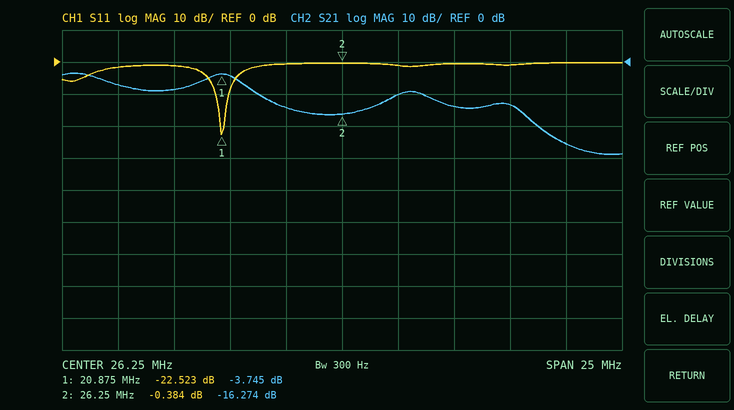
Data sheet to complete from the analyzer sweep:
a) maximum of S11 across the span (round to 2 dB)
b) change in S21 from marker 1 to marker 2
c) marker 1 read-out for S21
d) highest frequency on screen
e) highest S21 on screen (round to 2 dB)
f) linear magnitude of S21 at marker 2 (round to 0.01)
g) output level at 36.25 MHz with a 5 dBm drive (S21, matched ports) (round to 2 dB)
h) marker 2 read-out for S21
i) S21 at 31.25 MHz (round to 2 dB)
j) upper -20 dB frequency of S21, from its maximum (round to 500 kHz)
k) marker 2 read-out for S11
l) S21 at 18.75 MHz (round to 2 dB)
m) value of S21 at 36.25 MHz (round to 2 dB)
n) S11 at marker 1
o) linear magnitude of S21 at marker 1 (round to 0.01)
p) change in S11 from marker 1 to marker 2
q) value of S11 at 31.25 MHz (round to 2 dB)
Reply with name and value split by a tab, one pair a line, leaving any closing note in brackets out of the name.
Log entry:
maximum of S11 across the span	0 dB
change in S21 from marker 1 to marker 2	-12.529 dB
marker 1 read-out for S21	-3.745 dB
highest frequency on screen	38.75 MHz
highest S21 on screen	-4 dB
linear magnitude of S21 at marker 2	0.15
output level at 36.25 MHz with a 5 dBm drive (S21, matched ports)	-20 dBm
marker 2 read-out for S21	-16.274 dB
S21 at 31.25 MHz	-14 dB
upper -20 dB frequency of S21, from its maximum	35.5 MHz
marker 2 read-out for S11	-0.384 dB
S21 at 18.75 MHz	-8 dB
value of S21 at 36.25 MHz	-26 dB
S11 at marker 1	-22.523 dB
linear magnitude of S21 at marker 1	0.65
change in S11 from marker 1 to marker 2	22.139 dB
value of S11 at 31.25 MHz	0 dB
